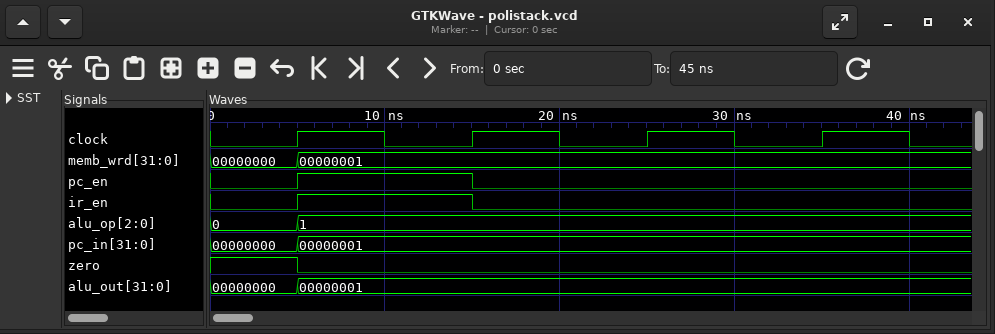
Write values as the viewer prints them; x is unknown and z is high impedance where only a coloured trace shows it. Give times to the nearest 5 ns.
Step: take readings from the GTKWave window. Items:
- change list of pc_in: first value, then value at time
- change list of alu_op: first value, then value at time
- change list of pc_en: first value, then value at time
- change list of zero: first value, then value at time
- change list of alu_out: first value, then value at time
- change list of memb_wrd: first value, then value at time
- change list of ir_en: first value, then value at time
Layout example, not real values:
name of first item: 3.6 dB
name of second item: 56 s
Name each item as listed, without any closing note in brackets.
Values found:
change list of pc_in: first value, then value at time: 00000000, 00000001 at 5 ns
change list of alu_op: first value, then value at time: 0, 1 at 5 ns
change list of pc_en: first value, then value at time: 0, 1 at 5 ns, 0 at 15 ns
change list of zero: first value, then value at time: 1, 0 at 5 ns
change list of alu_out: first value, then value at time: 00000000, 00000001 at 5 ns
change list of memb_wrd: first value, then value at time: 00000000, 00000001 at 5 ns
change list of ir_en: first value, then value at time: 0, 1 at 5 ns, 0 at 15 ns
